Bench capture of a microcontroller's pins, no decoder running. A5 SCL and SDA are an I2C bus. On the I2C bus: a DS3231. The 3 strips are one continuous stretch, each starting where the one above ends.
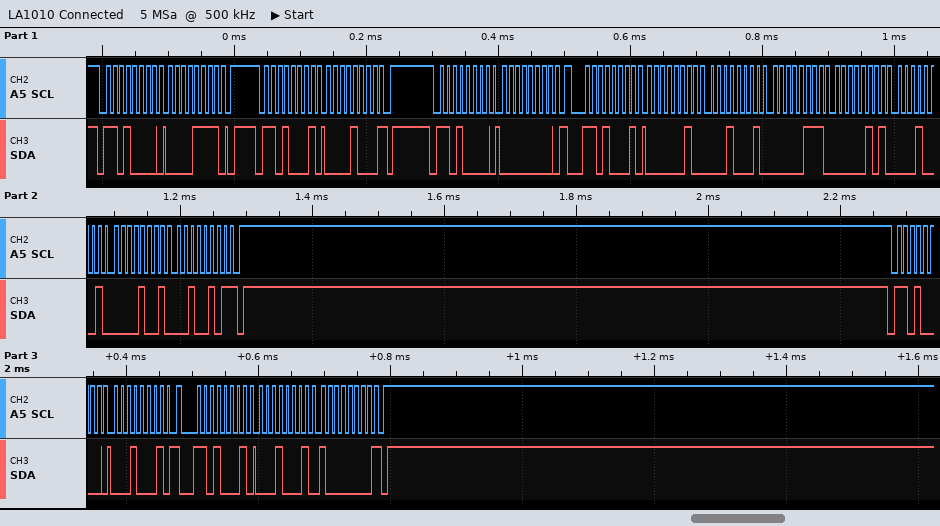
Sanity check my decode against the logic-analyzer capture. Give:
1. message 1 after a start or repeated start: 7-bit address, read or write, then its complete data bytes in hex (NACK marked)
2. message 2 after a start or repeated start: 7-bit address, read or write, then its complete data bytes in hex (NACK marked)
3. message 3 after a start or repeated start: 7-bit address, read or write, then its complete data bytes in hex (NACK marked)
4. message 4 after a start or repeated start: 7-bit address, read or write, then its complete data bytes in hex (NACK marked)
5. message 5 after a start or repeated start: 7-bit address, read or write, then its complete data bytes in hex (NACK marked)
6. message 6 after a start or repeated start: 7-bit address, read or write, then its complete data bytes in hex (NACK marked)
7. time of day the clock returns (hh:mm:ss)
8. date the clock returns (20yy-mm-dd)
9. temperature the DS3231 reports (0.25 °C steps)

0x68 write: 0F
0x68 read: 08 NACK
0x68 write: 00
0x68 read: 02 11 07 05 11 09 25 NACK
0x68 write: 11
0x68 read: 11 80 NACK
07:11:02
2025-09-11
17.50 °C
